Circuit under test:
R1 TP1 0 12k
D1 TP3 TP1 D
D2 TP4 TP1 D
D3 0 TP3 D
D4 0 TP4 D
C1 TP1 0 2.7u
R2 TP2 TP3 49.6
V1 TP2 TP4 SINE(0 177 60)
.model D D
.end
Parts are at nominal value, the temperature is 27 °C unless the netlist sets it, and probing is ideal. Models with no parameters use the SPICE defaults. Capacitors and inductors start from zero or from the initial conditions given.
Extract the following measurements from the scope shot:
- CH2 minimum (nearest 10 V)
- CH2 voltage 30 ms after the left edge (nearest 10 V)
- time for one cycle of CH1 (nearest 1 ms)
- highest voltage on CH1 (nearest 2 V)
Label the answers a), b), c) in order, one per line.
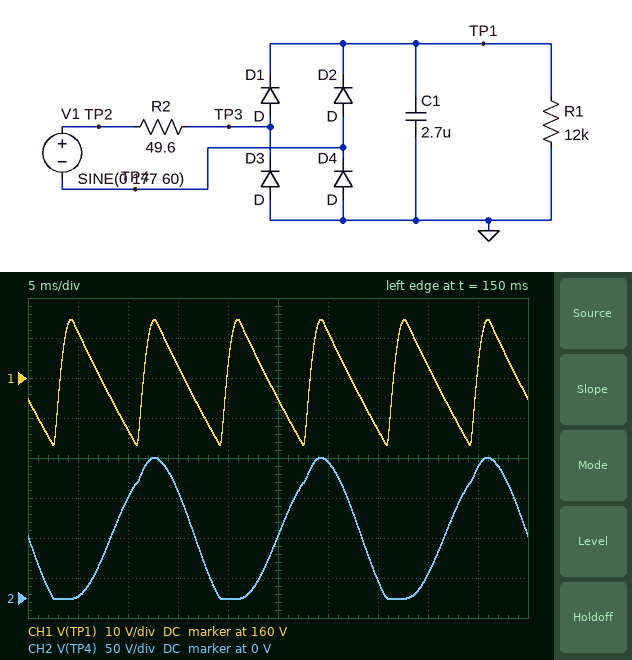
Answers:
a) 0 V
b) 170 V
c) 8 ms
d) 174 V
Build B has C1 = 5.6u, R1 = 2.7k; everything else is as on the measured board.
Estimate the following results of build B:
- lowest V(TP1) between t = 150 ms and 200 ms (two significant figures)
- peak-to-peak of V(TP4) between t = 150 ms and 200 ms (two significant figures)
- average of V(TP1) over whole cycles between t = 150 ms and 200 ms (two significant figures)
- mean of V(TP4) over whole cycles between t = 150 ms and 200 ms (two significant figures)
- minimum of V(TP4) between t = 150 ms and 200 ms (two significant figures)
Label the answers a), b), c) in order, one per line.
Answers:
a) 120 V
b) 170 V
c) 150 V
d) 73 V
e) -800 mV
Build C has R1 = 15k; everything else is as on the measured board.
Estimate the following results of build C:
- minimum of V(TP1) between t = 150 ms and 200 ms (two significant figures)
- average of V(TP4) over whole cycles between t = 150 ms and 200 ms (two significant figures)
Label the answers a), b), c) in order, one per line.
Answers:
a) 150 V
b) 81 V
